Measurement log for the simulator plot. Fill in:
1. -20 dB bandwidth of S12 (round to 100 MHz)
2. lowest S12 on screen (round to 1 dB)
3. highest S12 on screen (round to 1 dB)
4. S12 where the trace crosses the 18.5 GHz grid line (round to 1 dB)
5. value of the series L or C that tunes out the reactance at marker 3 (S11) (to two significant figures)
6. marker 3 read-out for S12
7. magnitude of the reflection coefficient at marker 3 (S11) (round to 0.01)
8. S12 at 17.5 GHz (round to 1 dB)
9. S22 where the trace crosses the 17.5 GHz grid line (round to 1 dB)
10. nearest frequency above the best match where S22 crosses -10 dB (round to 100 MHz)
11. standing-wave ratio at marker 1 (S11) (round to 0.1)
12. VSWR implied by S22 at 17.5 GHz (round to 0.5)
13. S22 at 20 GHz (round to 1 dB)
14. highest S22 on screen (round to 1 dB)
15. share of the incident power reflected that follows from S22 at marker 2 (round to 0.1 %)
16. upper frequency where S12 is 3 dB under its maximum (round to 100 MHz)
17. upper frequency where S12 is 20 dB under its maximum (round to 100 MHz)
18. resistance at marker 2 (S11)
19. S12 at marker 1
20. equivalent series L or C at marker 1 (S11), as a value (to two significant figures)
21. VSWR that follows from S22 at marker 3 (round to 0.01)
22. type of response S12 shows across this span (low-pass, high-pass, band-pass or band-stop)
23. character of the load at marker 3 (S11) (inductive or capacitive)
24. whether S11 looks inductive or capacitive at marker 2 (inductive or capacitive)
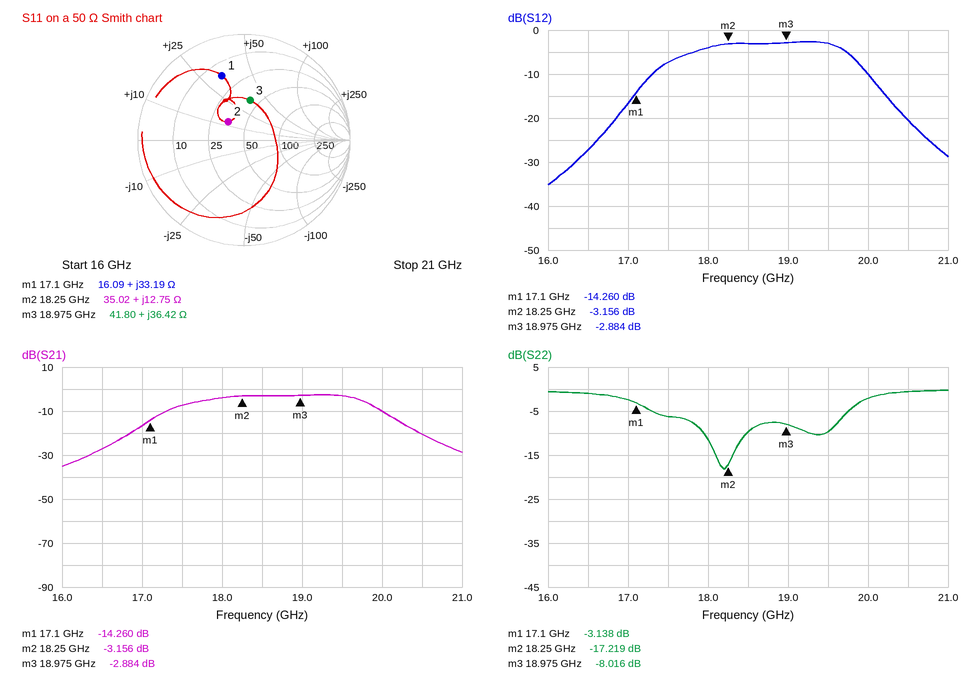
3.9 GHz
-35 dB
-3 dB
-3 dB
230 fF
-2.884 dB
0.38
-7 dB
-6 dB
18.5 GHz
4.6
3.0
-2 dB
0 dB
1.9 %
19.8 GHz
20.6 GHz
35.02 Ω
-14.260 dB
310 pH
2.32
band-pass
inductive
inductive
